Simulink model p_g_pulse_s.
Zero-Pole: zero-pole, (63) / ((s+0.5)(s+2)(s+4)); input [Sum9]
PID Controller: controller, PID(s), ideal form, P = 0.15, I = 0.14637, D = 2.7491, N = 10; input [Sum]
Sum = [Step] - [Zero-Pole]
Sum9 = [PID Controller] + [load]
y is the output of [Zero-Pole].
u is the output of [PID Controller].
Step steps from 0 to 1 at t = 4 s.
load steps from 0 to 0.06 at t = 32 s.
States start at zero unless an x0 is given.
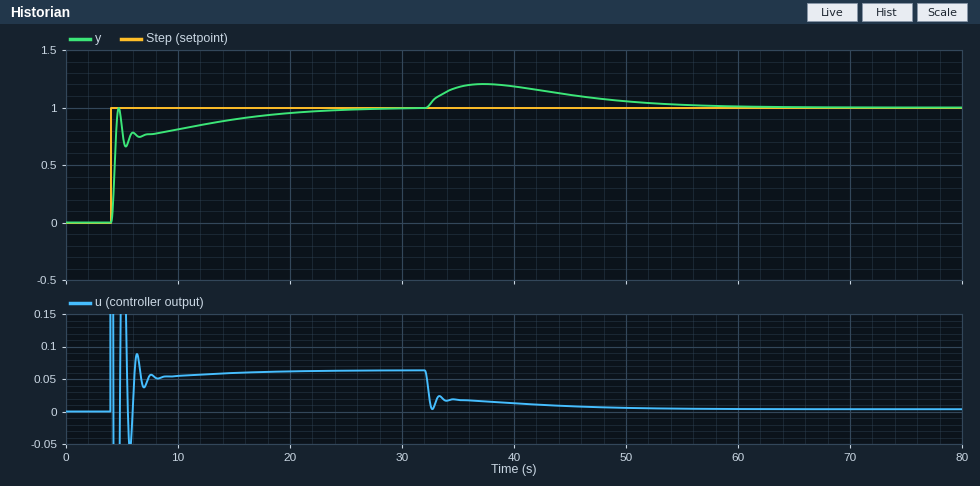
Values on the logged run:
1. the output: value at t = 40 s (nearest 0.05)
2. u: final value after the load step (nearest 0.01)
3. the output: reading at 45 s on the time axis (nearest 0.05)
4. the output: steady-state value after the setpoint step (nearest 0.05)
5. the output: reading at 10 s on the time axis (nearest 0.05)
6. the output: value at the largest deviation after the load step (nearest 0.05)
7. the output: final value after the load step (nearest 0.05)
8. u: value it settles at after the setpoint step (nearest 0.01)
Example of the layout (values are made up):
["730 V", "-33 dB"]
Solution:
["1.20", "0.00", "1.10", "1.00", "0.80", "1.20", "1.00", "0.06"]
